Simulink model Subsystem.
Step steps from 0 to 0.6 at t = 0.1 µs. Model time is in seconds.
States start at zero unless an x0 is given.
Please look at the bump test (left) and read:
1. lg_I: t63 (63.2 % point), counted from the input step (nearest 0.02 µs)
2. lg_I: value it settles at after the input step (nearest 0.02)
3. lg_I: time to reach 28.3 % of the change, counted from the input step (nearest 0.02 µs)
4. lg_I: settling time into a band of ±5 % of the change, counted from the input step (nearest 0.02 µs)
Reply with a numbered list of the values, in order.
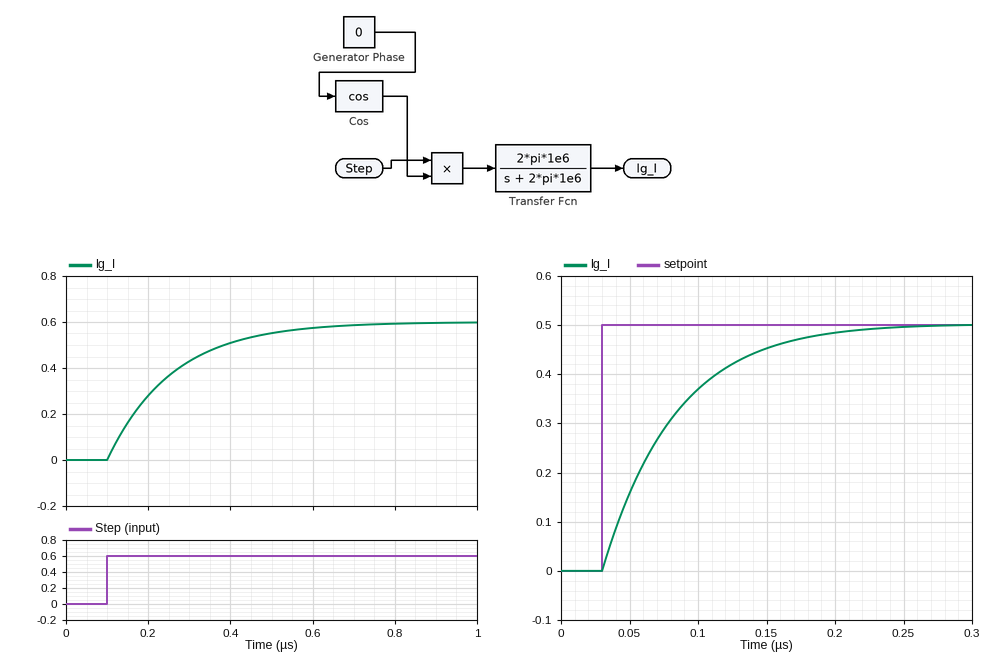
1. 0.16 µs
2. 0.60
3. 0.06 µs
4. 0.48 µs
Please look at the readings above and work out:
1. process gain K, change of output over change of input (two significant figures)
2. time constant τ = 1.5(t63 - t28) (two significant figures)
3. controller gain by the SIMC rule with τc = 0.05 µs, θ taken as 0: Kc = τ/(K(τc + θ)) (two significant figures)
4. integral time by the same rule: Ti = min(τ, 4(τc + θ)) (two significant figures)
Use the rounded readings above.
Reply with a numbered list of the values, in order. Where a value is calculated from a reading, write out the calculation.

1. (0.6 - 0) / 0.6 = 1.0
2. 1.5 × (0.16 - 0.06) = 0.15 µs
3. 0.15 / (1 × (0.05 + 0)) = 3.0
4. min(0.15, 4 × (0.05 + 0)) = 0.15 µs
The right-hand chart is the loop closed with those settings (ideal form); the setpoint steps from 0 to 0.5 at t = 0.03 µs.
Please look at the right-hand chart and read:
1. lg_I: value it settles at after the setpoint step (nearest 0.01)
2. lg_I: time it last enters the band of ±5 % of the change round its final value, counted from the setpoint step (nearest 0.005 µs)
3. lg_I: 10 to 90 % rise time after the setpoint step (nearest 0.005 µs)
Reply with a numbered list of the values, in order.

1. 0.50
2. 0.150 µs
3. 0.110 µs
